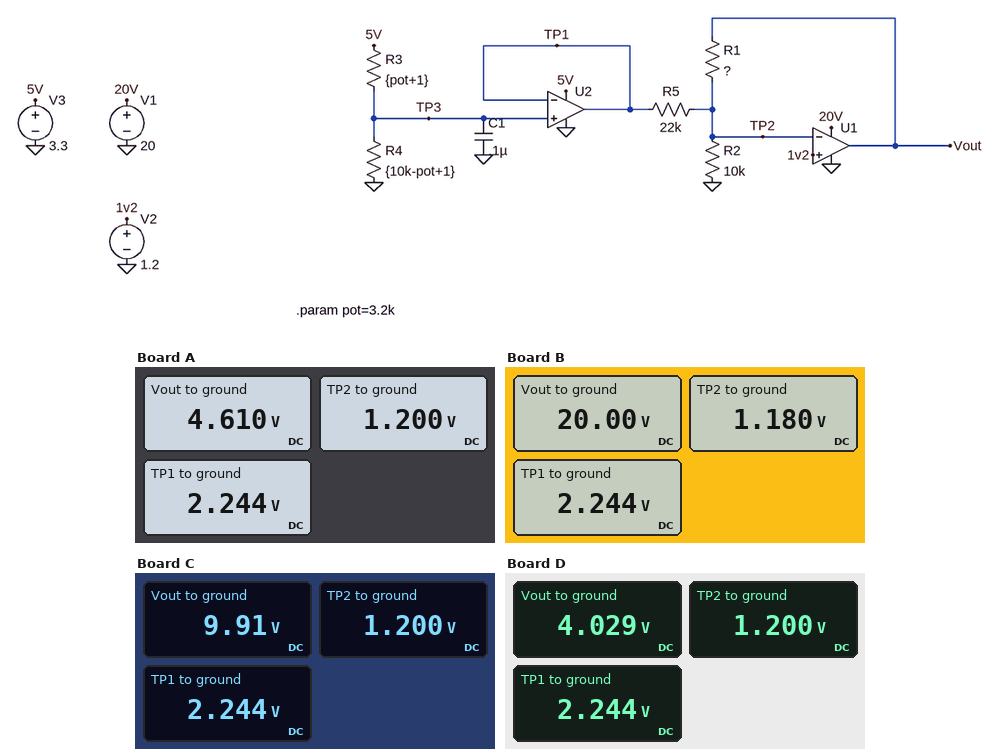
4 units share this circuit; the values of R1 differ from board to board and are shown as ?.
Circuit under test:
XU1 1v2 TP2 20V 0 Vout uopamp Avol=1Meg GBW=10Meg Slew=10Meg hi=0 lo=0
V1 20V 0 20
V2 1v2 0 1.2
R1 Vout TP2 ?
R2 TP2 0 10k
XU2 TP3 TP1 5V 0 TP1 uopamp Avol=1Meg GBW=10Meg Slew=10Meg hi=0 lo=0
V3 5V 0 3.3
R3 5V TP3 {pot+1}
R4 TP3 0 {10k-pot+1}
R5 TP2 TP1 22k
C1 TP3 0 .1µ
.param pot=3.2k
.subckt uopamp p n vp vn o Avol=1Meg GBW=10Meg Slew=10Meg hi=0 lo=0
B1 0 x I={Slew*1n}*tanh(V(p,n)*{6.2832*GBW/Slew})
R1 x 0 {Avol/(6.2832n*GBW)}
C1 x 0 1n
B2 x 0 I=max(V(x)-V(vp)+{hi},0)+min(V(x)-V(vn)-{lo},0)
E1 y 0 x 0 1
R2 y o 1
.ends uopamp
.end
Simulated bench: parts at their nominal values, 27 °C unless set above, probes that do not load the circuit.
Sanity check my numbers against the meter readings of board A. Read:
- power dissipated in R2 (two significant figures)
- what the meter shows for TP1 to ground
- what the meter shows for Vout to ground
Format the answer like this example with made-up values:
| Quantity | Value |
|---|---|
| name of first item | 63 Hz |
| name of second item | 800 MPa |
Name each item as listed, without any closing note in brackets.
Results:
| Quantity | Value |
|---|---|
| power dissipated in R2 | 140 µW |
| what the meter shows for TP1 to ground | 2.244 V |
| what the meter shows for Vout to ground | 4.610 V |
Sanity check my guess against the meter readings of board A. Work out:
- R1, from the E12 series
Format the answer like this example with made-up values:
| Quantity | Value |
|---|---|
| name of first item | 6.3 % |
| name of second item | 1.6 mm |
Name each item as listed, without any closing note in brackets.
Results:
| Quantity | Value |
|---|---|
| R1, from the E12 series | 47 kΩ |
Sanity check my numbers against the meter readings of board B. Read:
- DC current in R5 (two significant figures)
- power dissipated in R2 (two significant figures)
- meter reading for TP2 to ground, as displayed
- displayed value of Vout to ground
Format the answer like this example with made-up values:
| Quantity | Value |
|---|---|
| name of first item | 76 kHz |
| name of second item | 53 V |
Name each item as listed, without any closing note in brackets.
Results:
| Quantity | Value |
|---|---|
| DC current in R5 | 48 µA |
| power dissipated in R2 | 140 µW |
| meter reading for TP2 to ground, as displayed | 1.180 V |
| displayed value of Vout to ground | 20.00 V |
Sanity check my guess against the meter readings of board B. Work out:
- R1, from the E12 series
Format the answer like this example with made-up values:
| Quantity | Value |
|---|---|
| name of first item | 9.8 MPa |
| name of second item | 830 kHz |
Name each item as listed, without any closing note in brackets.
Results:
| Quantity | Value |
|---|---|
| R1, from the E12 series | 270 kΩ |
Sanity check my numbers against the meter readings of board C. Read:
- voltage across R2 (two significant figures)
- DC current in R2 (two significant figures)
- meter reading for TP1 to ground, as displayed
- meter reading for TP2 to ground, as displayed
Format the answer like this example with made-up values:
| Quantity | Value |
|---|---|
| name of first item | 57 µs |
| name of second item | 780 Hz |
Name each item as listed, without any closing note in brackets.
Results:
| Quantity | Value |
|---|---|
| voltage across R2 | 1.2 V |
| DC current in R2 | 120 µA |
| meter reading for TP1 to ground, as displayed | 2.244 V |
| meter reading for TP2 to ground, as displayed | 1.200 V |
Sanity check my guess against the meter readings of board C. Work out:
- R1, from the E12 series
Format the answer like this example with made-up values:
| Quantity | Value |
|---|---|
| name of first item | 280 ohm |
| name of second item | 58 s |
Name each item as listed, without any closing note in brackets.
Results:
| Quantity | Value |
|---|---|
| R1, from the E12 series | 120 kΩ |
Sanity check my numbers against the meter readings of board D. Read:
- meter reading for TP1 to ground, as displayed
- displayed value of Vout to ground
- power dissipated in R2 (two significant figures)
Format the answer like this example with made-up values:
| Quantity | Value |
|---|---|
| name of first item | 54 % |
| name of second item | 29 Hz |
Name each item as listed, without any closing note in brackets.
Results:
| Quantity | Value |
|---|---|
| meter reading for TP1 to ground, as displayed | 2.244 V |
| displayed value of Vout to ground | 4.029 V |
| power dissipated in R2 | 140 µW |
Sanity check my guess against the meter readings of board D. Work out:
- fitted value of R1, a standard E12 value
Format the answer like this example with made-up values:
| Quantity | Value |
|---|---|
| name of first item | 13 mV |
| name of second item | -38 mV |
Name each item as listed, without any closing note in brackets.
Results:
| Quantity | Value |
|---|---|
| fitted value of R1, a standard E12 value | 39 kΩ |
